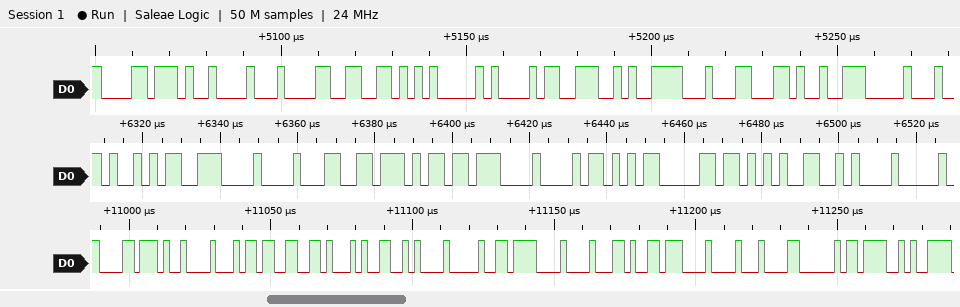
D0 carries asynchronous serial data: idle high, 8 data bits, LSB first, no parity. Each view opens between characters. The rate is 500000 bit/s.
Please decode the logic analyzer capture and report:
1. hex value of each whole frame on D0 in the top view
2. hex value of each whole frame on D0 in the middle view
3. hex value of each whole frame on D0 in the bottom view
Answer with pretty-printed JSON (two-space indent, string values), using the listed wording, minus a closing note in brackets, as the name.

{
  "hex value of each whole frame on D0 in the top view": "D8, 09, 84, 66, 05, A1, 4E, 1E, 8C, C9, 10",
  "hex value of each whole frame on D0 in the middle view": "A9, 0E, 88, 76, DB, 08, AB, B0, 95, 0A",
  "hex value of each whole frame on D0 in the bottom view": "D8, 09, B4, 66, 94, 0A, 90, 0F, 88, D9, 08, 84, A0, 4F"
}
